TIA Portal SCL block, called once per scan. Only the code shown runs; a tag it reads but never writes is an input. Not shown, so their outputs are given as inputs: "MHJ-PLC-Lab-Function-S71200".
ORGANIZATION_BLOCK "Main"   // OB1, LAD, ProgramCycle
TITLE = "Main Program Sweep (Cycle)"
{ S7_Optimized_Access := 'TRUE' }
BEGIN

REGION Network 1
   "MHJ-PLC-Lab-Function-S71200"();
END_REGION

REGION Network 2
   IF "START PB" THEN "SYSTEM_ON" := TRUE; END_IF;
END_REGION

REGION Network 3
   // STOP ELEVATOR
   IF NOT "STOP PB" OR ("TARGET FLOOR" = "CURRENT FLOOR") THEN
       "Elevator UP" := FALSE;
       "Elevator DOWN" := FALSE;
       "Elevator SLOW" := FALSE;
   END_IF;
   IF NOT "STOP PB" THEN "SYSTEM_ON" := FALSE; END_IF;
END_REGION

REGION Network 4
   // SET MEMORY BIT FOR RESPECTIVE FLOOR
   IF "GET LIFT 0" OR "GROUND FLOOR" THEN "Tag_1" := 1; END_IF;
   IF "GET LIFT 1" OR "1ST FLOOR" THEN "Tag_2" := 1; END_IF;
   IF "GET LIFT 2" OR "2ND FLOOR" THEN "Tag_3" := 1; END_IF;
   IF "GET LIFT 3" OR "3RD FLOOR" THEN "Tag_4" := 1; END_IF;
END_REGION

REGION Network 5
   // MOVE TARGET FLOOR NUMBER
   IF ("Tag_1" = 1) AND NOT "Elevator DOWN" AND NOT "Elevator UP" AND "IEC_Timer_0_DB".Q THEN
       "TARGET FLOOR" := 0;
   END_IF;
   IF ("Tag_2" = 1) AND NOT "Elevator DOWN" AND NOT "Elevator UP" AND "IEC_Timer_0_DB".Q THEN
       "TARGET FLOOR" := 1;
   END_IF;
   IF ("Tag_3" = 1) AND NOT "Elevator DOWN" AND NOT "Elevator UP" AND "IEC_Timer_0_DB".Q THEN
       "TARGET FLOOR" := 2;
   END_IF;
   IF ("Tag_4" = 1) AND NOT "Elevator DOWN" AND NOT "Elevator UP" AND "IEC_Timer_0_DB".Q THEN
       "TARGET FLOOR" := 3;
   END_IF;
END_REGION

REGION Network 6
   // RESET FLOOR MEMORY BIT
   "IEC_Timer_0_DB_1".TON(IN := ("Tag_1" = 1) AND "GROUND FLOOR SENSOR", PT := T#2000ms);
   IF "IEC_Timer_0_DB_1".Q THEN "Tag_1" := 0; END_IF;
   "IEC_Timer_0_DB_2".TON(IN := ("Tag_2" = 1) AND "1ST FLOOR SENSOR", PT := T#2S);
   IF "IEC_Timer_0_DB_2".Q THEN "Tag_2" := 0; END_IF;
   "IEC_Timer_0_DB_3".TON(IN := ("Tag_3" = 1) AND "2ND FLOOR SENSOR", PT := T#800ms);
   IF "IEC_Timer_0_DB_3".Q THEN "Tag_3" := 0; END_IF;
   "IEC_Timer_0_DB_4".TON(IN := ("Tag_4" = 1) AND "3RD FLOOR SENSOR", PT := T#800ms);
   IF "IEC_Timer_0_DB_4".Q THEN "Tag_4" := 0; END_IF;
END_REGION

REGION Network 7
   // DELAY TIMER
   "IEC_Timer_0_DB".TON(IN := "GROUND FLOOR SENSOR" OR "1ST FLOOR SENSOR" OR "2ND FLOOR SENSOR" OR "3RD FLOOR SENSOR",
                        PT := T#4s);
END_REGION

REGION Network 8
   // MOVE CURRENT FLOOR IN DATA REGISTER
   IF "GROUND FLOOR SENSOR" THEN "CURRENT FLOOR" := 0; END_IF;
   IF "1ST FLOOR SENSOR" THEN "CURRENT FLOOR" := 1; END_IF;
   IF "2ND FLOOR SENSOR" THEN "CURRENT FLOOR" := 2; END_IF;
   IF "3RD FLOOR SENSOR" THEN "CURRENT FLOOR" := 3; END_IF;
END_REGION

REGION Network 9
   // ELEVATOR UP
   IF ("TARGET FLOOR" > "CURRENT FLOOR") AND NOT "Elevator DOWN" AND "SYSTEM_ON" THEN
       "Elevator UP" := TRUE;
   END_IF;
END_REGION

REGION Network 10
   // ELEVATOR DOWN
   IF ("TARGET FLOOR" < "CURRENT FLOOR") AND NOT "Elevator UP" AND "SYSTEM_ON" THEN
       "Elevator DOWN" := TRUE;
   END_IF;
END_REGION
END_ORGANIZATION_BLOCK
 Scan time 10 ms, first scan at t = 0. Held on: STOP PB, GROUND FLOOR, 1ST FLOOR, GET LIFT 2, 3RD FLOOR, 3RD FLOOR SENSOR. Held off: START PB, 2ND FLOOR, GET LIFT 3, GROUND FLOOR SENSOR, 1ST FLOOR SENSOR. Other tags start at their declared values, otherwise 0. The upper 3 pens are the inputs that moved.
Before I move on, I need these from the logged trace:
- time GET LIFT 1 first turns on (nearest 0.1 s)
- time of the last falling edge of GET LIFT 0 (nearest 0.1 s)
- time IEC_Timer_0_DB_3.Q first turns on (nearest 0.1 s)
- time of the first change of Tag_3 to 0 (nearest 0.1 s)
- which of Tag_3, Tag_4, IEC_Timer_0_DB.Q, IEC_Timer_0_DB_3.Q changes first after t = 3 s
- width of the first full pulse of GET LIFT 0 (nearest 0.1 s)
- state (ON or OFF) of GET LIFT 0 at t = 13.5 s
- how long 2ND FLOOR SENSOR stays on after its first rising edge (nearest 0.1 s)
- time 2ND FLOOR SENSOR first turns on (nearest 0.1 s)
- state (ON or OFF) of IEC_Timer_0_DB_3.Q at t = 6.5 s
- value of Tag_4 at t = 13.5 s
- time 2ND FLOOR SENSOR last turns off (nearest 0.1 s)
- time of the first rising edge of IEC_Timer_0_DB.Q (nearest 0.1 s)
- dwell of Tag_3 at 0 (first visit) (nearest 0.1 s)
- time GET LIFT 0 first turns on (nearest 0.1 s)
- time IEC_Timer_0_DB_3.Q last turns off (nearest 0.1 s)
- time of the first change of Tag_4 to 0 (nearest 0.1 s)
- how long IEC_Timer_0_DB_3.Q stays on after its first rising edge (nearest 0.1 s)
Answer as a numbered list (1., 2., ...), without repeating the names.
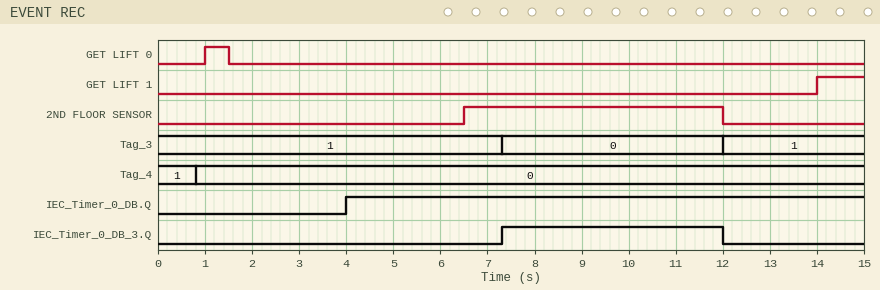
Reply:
1. 14.0 s
2. 1.5 s
3. 7.3 s
4. 7.3 s
5. IEC_Timer_0_DB.Q
6. 0.5 s
7. OFF
8. 5.5 s
9. 6.5 s
10. OFF
11. 0
12. 12.0 s
13. 4.0 s
14. 4.7 s
15. 1.0 s
16. 12.0 s
17. 0.8 s
18. 4.7 s
